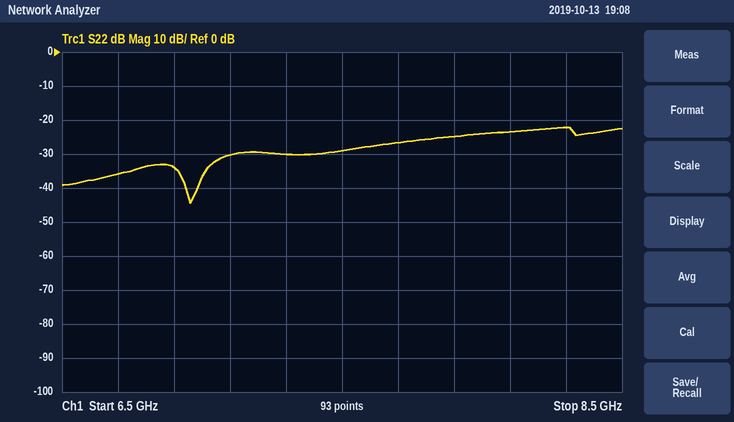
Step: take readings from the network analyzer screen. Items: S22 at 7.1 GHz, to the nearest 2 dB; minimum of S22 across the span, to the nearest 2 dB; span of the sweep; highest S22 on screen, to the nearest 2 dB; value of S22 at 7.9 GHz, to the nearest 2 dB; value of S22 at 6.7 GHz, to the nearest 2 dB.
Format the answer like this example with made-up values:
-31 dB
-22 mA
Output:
-30 dB
-44 dB
2 GHz
-22 dB
-24 dB
-36 dB
